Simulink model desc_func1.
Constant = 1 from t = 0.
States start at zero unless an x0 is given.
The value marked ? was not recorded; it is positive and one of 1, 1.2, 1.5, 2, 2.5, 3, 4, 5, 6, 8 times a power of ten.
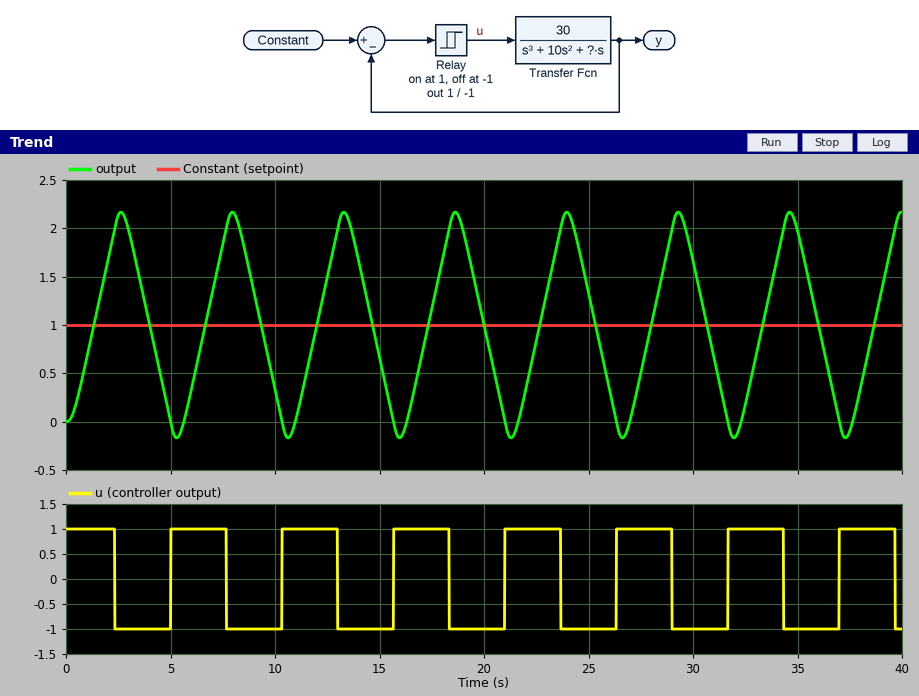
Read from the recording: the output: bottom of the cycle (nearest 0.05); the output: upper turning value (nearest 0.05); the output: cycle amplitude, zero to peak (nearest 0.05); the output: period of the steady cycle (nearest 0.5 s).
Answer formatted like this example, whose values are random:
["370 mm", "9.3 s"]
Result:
["-0.15", "2.15", "1.15", "5.5 s"]
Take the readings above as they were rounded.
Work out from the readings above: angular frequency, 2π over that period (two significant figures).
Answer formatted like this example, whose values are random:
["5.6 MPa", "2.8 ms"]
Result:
["1.1 rad/s"]
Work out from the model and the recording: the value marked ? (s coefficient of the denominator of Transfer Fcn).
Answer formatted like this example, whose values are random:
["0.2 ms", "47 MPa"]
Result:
["30"]
